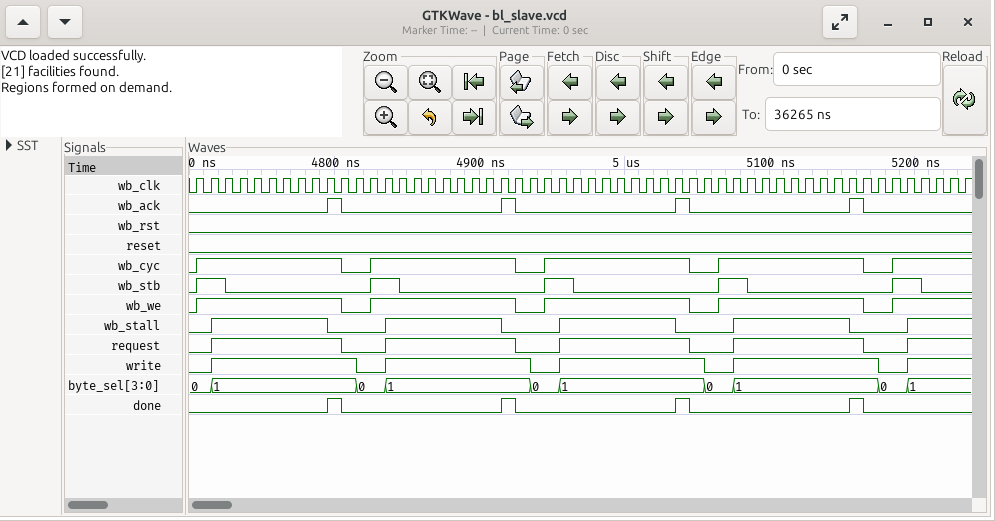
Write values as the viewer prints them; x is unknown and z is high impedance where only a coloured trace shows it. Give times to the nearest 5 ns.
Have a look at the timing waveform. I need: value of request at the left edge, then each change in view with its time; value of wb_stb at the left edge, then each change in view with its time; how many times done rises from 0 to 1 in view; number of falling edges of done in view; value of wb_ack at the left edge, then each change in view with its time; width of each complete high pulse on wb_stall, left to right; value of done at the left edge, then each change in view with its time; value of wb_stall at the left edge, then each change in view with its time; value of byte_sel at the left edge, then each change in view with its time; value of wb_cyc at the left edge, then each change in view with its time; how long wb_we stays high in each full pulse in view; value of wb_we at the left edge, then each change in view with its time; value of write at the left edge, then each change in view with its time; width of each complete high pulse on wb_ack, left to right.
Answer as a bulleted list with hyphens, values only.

- 0, 1 at 4715 ns, 0 at 4805 ns, 1 at 4835 ns, 0 at 4925 ns, 1 at 4955 ns, 0 at 5045 ns, 1 at 5075 ns, 0 at 5165 ns, 1 at 5195 ns
- 0, 1 at 4705 ns, 0 at 4725 ns, 1 at 4825 ns, 0 at 4845 ns, 1 at 4945 ns, 0 at 4965 ns, 1 at 5065 ns, 0 at 5085 ns, 1 at 5185 ns, 0 at 5205 ns
- 4
- 4
- 0, 1 at 4795 ns, 0 at 4805 ns, 1 at 4915 ns, 0 at 4925 ns, 1 at 5035 ns, 0 at 5045 ns, 1 at 5155 ns, 0 at 5165 ns
- 80 ns, 80 ns, 80 ns, 80 ns
- 0, 1 at 4795 ns, 0 at 4805 ns, 1 at 4915 ns, 0 at 4925 ns, 1 at 5035 ns, 0 at 5045 ns, 1 at 5155 ns, 0 at 5165 ns
- 0, 1 at 4715 ns, 0 at 4795 ns, 1 at 4835 ns, 0 at 4915 ns, 1 at 4955 ns, 0 at 5035 ns, 1 at 5075 ns, 0 at 5155 ns, 1 at 5195 ns
- 0, 1 at 4715 ns, 0 at 4815 ns, 1 at 4835 ns, 0 at 4935 ns, 1 at 4955 ns, 0 at 5055 ns, 1 at 5075 ns, 0 at 5175 ns, 1 at 5195 ns
- 0, 1 at 4705 ns, 0 at 4805 ns, 1 at 4825 ns, 0 at 4925 ns, 1 at 4945 ns, 0 at 5045 ns, 1 at 5065 ns, 0 at 5165 ns, 1 at 5185 ns
- 100 ns, 100 ns, 100 ns, 100 ns
- 0, 1 at 4705 ns, 0 at 4805 ns, 1 at 4825 ns, 0 at 4925 ns, 1 at 4945 ns, 0 at 5045 ns, 1 at 5065 ns, 0 at 5165 ns, 1 at 5185 ns
- 0, 1 at 4715 ns, 0 at 4815 ns, 1 at 4835 ns, 0 at 4935 ns, 1 at 4955 ns, 0 at 5055 ns, 1 at 5075 ns, 0 at 5175 ns, 1 at 5195 ns
- 10 ns, 10 ns, 10 ns, 10 ns
